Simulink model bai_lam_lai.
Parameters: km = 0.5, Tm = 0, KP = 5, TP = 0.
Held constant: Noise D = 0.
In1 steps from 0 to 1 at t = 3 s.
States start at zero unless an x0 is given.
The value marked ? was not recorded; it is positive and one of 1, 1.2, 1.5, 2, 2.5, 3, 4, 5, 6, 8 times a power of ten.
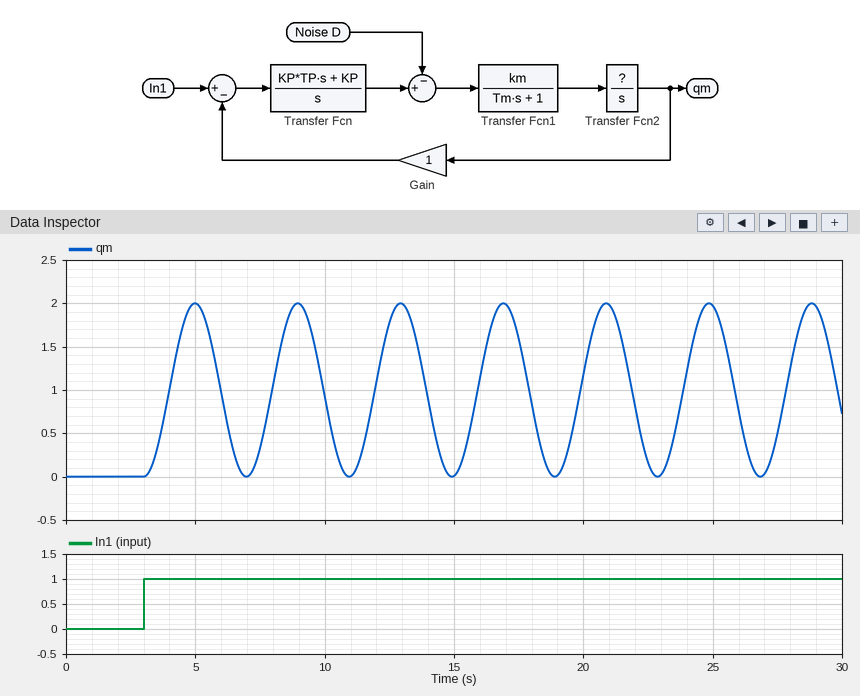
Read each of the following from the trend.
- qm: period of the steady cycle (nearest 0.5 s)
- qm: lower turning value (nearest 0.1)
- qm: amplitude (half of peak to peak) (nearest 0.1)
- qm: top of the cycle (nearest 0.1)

4.0 s
0.0
1.0
2.0
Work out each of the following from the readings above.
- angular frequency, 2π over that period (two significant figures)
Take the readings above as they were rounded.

1.6 rad/s
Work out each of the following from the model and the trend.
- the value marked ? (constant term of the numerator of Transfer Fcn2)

1
